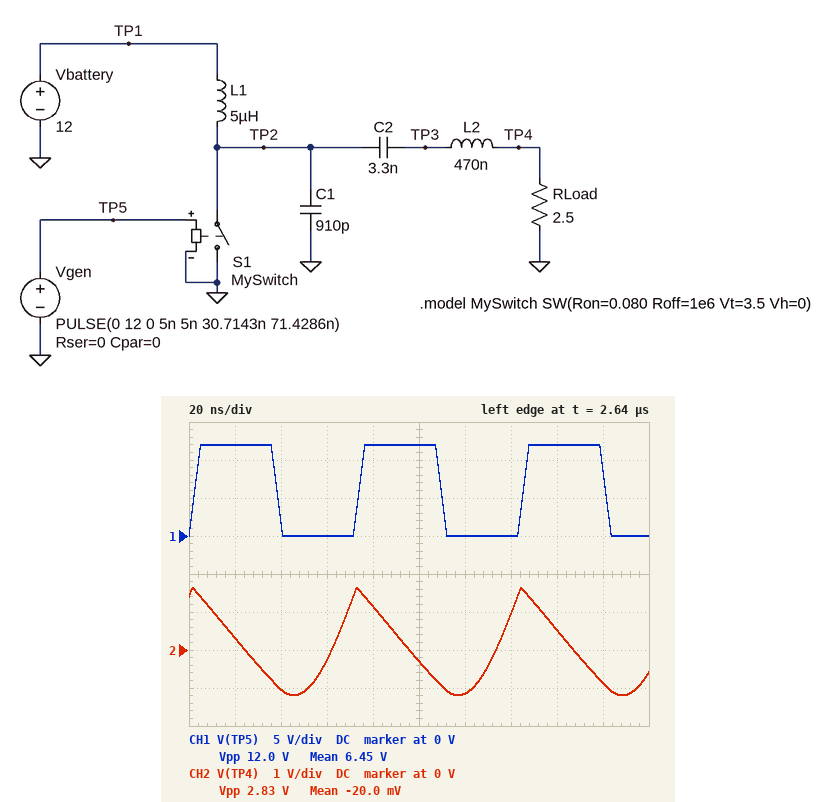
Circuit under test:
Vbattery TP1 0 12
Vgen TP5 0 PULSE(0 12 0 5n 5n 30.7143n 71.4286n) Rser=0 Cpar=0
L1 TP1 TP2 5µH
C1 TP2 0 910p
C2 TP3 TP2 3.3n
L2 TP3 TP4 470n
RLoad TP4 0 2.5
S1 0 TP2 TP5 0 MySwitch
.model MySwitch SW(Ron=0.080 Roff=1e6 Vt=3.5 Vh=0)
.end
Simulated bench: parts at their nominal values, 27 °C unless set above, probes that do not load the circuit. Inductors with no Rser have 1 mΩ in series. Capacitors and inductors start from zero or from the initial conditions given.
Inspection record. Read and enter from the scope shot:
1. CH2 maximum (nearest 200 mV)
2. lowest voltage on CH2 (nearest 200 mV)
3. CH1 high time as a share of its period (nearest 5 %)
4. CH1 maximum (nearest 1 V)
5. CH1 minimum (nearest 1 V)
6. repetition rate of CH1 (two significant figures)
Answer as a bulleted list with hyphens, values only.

- 1.6 V
- -1.2 V
- 50 %
- 12 V
- 0 V
- 14 MHz
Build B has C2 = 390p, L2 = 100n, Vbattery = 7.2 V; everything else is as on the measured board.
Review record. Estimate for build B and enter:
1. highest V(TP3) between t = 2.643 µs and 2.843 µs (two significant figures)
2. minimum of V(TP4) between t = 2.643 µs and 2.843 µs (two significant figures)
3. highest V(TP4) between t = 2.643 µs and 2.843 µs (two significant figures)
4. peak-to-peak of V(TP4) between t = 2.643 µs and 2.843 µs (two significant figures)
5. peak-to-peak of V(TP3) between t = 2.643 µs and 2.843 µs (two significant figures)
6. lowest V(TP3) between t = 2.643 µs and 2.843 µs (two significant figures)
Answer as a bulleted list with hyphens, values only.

- 26 V
- -4.7 V
- 3.6 V
- 8.3 V
- 60 V
- -34 V
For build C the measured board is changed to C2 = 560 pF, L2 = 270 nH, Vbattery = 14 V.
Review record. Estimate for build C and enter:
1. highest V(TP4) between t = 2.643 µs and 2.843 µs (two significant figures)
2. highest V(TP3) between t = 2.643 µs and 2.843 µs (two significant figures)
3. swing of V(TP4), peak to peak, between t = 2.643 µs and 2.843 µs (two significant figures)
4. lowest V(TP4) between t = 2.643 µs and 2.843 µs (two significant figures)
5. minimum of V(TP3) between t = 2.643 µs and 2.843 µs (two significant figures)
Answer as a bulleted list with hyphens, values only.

- 13 V
- 130 V
- 25 V
- -12 V
- -110 V
